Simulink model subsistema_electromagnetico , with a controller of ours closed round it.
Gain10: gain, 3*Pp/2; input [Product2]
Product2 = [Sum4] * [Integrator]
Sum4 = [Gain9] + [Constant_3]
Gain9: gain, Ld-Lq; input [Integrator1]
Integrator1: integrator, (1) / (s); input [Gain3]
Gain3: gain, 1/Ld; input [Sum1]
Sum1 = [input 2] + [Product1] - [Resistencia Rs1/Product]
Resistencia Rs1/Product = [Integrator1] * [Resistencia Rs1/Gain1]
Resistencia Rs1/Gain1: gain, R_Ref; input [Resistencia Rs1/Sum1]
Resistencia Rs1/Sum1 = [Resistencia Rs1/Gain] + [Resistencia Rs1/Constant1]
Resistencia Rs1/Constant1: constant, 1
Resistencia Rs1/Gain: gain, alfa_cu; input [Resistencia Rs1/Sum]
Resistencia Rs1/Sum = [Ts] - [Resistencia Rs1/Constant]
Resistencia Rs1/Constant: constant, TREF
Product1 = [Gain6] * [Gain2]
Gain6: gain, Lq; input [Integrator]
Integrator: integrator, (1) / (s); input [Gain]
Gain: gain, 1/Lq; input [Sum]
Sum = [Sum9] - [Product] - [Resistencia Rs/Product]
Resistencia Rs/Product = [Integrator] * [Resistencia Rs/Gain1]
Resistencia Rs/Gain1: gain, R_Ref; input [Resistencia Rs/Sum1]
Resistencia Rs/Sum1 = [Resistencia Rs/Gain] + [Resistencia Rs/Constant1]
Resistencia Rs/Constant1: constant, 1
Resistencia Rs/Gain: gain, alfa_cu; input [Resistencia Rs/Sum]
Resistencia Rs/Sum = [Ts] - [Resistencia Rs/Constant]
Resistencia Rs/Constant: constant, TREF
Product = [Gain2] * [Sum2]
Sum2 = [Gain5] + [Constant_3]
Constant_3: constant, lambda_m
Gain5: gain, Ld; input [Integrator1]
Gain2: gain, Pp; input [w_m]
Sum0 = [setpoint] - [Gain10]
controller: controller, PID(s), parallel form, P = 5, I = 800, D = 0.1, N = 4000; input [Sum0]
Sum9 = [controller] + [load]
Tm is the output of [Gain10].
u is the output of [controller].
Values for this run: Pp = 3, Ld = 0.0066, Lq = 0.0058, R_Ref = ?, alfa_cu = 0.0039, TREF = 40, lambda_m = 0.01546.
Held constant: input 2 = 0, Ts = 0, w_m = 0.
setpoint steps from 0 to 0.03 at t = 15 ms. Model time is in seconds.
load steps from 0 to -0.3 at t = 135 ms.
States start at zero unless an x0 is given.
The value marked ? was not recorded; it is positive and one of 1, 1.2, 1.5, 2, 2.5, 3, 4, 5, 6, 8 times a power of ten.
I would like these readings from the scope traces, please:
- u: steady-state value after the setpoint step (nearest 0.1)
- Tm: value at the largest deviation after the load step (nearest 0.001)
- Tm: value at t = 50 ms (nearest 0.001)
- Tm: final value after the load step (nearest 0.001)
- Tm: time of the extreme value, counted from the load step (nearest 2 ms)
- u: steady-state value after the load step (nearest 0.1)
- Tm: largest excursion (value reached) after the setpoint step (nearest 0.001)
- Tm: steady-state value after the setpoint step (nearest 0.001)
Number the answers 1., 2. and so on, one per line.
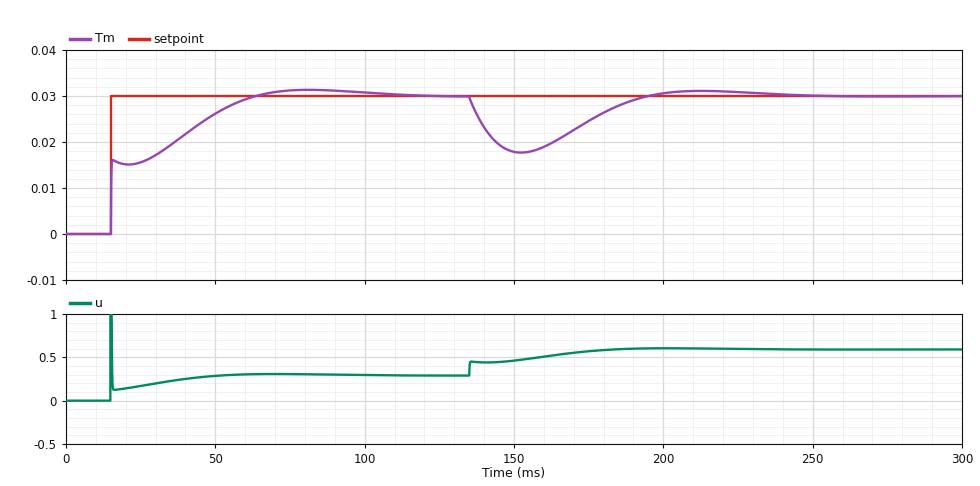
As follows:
1. 0.3
2. 0.018
3. 0.026
4. 0.030
5. 18 ms
6. 0.6
7. 0.031
8. 0.030
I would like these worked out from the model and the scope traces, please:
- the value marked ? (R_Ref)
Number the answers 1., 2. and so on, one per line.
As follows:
1. 0.8
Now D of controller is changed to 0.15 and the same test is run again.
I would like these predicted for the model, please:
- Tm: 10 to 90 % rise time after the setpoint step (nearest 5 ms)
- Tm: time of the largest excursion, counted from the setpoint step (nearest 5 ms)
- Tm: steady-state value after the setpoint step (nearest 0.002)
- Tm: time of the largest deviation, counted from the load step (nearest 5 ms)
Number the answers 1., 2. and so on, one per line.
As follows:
1. 40 ms
2. 75 ms
3. 0.030
4. 20 ms
